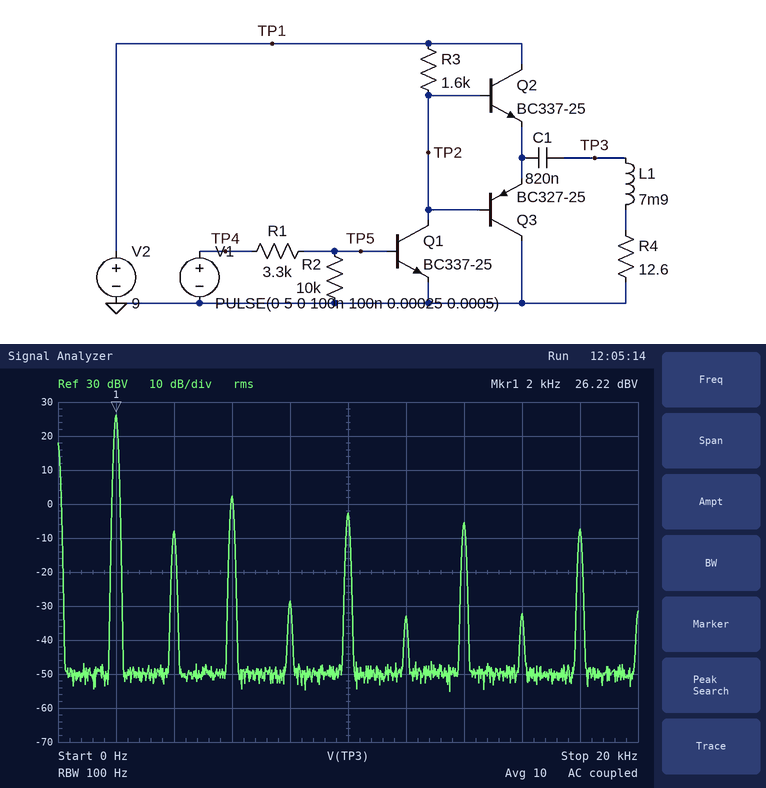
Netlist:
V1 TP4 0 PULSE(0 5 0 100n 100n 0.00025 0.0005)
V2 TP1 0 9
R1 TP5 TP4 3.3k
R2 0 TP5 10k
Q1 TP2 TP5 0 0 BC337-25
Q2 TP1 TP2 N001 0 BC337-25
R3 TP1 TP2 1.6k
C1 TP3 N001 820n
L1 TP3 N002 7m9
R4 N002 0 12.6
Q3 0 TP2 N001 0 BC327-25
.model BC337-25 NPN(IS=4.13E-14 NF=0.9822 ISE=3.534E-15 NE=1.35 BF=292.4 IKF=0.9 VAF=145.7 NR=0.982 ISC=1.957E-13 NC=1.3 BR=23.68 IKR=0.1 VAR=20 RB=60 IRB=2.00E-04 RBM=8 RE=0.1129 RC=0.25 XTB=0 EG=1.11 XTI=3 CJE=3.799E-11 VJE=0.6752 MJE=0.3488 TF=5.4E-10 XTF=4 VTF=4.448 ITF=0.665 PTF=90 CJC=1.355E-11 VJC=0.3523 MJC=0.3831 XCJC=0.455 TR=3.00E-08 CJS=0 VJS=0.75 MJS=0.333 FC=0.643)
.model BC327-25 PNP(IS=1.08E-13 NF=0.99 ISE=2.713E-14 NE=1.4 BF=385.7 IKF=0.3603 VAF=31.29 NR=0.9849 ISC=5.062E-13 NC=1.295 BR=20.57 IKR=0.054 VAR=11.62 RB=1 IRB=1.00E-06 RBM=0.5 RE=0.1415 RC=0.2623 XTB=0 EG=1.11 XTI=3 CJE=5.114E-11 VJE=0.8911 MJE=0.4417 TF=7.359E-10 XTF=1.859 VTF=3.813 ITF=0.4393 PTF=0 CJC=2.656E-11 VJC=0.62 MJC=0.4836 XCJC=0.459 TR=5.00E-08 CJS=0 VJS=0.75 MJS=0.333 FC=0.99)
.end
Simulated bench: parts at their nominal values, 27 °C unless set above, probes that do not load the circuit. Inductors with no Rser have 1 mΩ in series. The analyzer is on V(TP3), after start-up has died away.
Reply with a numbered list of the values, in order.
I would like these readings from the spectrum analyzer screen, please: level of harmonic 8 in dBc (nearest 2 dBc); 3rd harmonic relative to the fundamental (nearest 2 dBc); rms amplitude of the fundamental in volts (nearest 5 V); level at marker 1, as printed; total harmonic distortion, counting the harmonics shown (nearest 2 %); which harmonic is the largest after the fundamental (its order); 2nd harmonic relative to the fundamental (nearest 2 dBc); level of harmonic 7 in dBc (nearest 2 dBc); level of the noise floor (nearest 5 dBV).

1. -58 dBc
2. -24 dBc
3. 20 V
4. 26.22 dBV
5. 8 %
6. 3
7. -34 dBc
8. -32 dBc
9. -50 dBV
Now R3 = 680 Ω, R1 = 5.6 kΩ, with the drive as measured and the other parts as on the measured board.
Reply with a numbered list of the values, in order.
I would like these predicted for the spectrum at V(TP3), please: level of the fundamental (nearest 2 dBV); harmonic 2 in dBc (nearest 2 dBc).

1. 28 dBV
2. -42 dBc
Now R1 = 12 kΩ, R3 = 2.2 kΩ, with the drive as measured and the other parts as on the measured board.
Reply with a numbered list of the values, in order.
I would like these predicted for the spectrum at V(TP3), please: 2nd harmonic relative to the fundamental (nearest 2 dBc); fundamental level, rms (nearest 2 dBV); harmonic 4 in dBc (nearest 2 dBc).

1. -32 dBc
2. 26 dBV
3. -50 dBc
